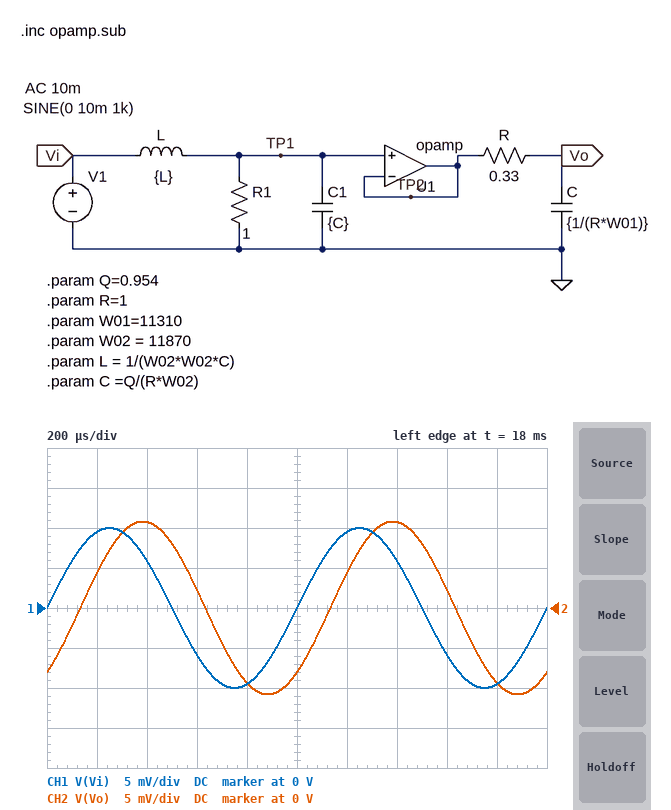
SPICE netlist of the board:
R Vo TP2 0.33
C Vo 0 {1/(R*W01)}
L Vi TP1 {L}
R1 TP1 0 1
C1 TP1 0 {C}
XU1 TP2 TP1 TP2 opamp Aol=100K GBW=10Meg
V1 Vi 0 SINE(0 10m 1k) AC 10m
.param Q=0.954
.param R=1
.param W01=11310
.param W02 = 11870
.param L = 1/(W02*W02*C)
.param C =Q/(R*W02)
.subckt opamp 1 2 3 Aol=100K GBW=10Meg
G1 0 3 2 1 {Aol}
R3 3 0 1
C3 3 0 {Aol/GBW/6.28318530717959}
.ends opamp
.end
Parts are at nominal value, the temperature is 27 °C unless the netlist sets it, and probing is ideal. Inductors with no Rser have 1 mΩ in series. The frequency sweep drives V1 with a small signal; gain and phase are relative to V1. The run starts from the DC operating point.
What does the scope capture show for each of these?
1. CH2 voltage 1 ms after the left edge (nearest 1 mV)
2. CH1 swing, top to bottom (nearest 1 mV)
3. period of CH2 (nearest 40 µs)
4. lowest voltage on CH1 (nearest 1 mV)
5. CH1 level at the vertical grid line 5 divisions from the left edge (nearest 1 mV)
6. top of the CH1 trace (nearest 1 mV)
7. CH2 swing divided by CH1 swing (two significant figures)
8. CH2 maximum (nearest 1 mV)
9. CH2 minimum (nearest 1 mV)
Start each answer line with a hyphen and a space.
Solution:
- -8 mV
- 20 mV
- 1.00 ms
- -10 mV
- 0 V
- 10 mV
- 1.1
- 11 mV
- -11 mV
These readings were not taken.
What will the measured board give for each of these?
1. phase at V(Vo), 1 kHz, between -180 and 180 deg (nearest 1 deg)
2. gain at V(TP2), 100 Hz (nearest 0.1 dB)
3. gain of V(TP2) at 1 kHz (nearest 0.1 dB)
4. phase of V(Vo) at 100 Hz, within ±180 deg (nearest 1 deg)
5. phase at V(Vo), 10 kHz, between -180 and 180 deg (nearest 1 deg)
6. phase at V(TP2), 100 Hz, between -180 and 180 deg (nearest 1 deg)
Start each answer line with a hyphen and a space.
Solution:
- -48 deg
- 0 dB
- 0.8 dB
- -4 deg
- 130 deg
- -3 deg
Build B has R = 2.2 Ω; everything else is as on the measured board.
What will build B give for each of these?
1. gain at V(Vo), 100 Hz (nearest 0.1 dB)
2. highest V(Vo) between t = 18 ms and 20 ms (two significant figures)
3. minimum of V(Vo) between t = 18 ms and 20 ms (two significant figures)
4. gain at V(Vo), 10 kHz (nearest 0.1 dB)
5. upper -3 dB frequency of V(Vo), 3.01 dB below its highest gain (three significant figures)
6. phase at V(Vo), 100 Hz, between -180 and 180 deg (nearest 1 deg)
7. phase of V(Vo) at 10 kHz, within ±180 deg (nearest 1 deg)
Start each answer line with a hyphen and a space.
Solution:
- -0.1 dB
- 7.0 mV
- -7.0 mV
- -50.6 dB
- 969 Hz
- -10 deg
- 106 deg
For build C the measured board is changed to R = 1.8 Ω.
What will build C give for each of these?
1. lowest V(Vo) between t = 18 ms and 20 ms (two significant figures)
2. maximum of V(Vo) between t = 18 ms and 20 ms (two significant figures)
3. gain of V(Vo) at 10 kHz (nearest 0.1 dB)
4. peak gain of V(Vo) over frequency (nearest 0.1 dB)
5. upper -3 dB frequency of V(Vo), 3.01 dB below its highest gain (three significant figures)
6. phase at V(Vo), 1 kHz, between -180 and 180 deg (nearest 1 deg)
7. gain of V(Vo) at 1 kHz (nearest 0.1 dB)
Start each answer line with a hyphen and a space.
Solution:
- -7.8 mV
- 7.8 mV
- -48.9 dB
- 0 dB
- 1.23 kHz
- -83 deg
- -2.2 dB
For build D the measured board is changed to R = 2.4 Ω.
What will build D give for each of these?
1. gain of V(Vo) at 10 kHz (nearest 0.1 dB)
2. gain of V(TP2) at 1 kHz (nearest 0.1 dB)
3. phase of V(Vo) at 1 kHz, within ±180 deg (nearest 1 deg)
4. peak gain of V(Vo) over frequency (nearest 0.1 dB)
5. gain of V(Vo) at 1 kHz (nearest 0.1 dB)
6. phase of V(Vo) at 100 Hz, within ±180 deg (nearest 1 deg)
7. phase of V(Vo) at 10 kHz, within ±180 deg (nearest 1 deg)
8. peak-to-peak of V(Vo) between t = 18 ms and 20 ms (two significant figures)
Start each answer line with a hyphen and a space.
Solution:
- -51.3 dB
- 0.8 dB
- -91 deg
- 0 dB
- -3.6 dB
- -11 deg
- 106 deg
- 13 mV
